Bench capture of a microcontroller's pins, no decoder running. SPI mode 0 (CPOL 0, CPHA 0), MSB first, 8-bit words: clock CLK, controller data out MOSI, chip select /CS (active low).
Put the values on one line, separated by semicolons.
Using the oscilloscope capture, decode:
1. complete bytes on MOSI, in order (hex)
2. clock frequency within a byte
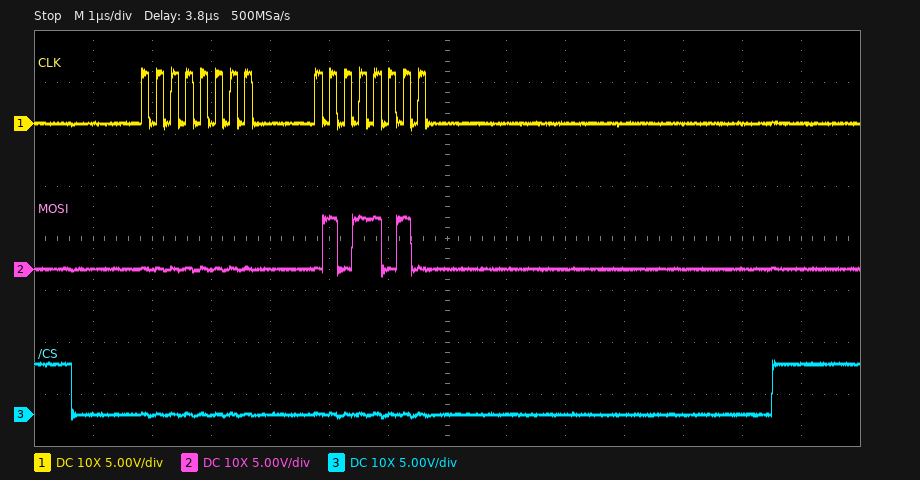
0x00 0x5A; 4 MHz
